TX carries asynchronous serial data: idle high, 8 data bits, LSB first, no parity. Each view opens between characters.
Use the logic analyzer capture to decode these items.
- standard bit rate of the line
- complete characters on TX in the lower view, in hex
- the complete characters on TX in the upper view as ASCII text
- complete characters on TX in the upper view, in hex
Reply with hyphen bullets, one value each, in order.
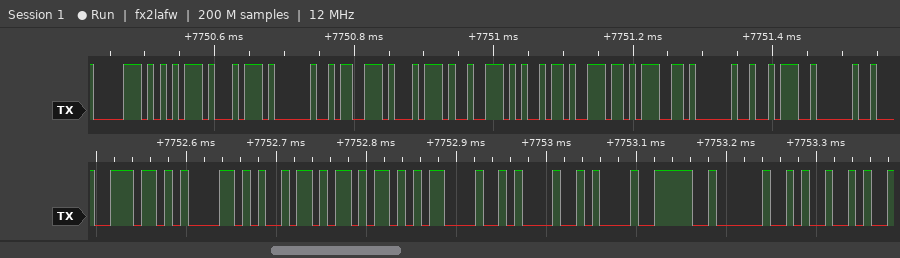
- 115200 baud
- 6E, 61, 69, 6B, 0D, 0A, 0A, 3E, 20, 49
- "put string : "
- 70, 75, 74, 20, 73, 74, 72, 69, 6E, 67, 20, 3A, 20
